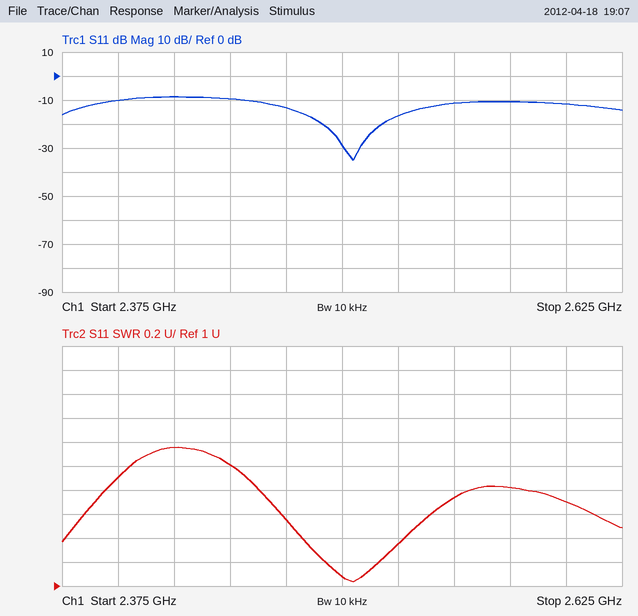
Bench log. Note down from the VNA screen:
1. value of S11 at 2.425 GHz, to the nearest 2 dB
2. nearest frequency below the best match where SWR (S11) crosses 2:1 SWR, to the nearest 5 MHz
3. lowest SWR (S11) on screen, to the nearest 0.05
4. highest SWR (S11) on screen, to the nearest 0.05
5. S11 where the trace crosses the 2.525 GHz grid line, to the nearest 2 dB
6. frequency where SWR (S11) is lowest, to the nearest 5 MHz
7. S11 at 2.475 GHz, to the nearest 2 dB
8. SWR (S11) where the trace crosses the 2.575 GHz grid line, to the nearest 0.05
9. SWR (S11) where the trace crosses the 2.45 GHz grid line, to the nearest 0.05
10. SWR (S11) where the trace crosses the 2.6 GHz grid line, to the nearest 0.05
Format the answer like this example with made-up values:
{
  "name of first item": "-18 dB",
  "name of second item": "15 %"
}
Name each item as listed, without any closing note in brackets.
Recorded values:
{
  "value of S11 at 2.425 GHz, to the nearest 2 dB": "-8 dB",
  "nearest frequency below the best match where SWR (S11) crosses 2:1 SWR, to the nearest 5 MHz": "2.450 GHz",
  "lowest SWR (S11) on screen, to the nearest 0.05": "1.05",
  "highest SWR (S11) on screen, to the nearest 0.05": "2.15",
  "S11 where the trace crosses the 2.525 GHz grid line, to the nearest 2 dB": "-16 dB",
  "frequency where SWR (S11) is lowest, to the nearest 5 MHz": "2.505 GHz",
  "S11 at 2.475 GHz, to the nearest 2 dB": "-14 dB",
  "SWR (S11) where the trace crosses the 2.575 GHz grid line, to the nearest 0.05": "1.80",
  "SWR (S11) where the trace crosses the 2.45 GHz grid line, to the nearest 0.05": "2.00",
  "SWR (S11) where the trace crosses the 2.6 GHz grid line, to the nearest 0.05": "1.70"
}
